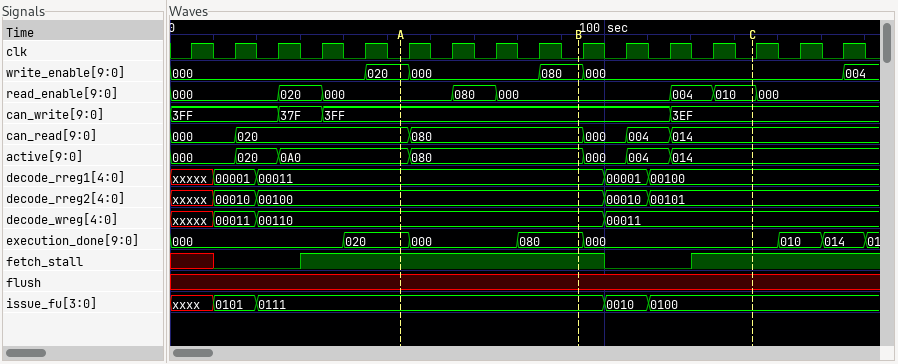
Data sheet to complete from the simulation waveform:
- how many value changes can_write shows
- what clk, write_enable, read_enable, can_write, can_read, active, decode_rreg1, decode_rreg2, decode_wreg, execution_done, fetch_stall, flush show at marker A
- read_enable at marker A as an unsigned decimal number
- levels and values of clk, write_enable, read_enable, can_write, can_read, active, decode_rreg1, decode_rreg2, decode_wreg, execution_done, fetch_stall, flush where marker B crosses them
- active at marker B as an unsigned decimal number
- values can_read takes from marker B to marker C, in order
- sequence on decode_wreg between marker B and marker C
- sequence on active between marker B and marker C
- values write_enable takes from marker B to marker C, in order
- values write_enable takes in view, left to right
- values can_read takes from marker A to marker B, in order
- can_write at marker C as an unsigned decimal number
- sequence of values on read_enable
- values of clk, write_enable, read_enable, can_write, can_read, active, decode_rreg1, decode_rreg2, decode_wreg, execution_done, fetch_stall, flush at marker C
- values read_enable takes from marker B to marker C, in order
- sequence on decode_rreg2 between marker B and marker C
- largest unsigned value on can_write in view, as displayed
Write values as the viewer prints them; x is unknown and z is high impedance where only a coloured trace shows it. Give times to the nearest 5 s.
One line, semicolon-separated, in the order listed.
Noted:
3; clk=0, write_enable=020, read_enable=000, can_write=3FF, can_read=020, active=0A0, decode_rreg1=00011, decode_rreg2=00100, decode_wreg=00110, execution_done=020, fetch_stall=1, flush=x; 0; clk=0, write_enable=080, read_enable=000, can_write=3FF, can_read=080, active=080, decode_rreg1=00011, decode_rreg2=00100, decode_wreg=00110, execution_done=080, fetch_stall=1, flush=x; 128; 080, 000, 004, 014; 00110, 00011; 080, 000, 004, 014; 080, 000; 000, 020, 000, 080, 000, 004; 020, 080; 1007; 000, 020, 000, 080, 000, 004, 010, 000; clk=0, write_enable=000, read_enable=010, can_write=3EF, can_read=014, active=014, decode_rreg1=00100, decode_rreg2=00101, decode_wreg=00011, execution_done=000, fetch_stall=1, flush=x; 000, 004, 010; 00100, 00010, 00101; 3FF
